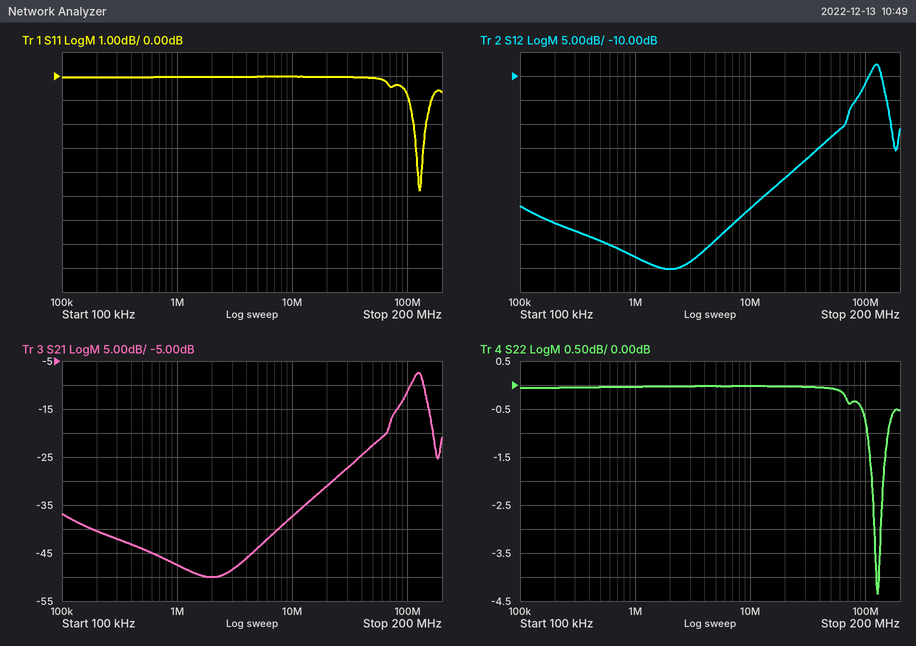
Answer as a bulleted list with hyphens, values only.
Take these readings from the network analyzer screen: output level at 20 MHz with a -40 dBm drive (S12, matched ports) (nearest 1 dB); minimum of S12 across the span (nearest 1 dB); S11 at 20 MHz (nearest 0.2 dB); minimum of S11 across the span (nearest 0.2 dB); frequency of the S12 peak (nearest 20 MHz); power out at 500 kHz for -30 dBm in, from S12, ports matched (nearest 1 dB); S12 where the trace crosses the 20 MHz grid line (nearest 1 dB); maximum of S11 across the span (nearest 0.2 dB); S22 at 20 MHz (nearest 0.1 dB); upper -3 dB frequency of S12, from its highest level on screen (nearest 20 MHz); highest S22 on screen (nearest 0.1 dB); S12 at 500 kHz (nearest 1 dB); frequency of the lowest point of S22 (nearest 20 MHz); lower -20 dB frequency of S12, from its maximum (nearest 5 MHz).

- -71 dBm
- -50 dB
- 0.0 dB
- -4.8 dB
- 120 MHz
- -74 dBm
- -31 dB
- 0.0 dB
- 0.0 dB
- 140 MHz
- 0.0 dB
- -44 dB
- 120 MHz
- 30 MHz
